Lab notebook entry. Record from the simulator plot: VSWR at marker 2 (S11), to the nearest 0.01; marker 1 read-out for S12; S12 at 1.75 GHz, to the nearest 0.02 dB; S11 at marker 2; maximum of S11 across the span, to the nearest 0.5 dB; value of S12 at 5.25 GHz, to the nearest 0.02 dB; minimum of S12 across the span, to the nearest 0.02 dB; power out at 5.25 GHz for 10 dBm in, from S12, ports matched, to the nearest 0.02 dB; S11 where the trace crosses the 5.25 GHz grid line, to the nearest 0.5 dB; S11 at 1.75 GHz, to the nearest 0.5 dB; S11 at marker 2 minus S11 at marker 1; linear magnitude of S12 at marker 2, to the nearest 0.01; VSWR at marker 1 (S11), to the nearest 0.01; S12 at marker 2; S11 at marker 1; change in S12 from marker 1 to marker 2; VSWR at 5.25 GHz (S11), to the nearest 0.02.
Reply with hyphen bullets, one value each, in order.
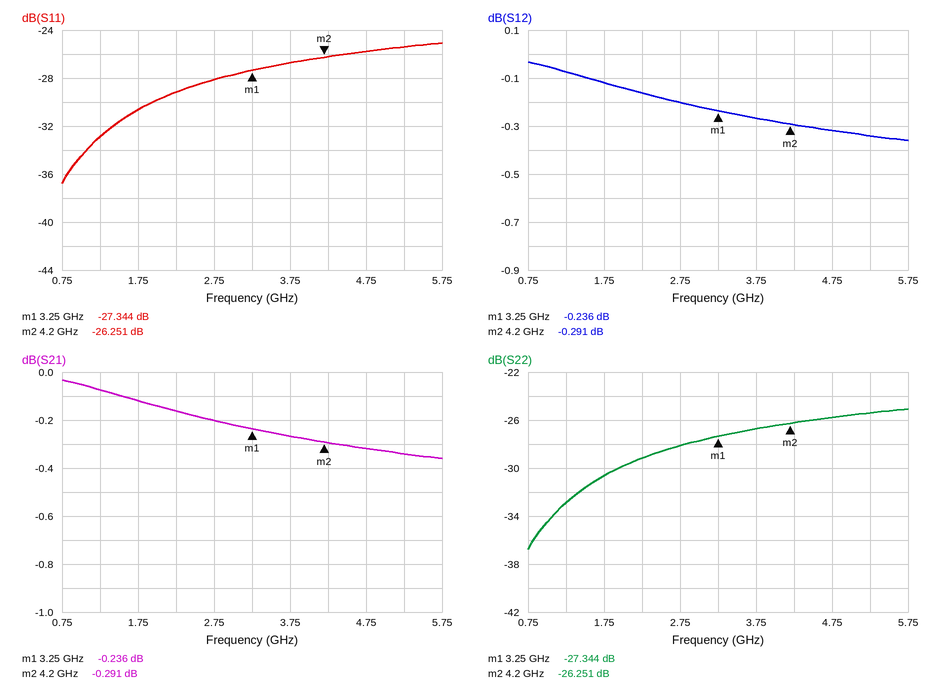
- 1.10
- -0.236 dB
- -0.12 dB
- -26.251 dB
- -25.0 dB
- -0.34 dB
- -0.36 dB
- 9.66 dBm
- -25.5 dB
- -30.5 dB
- 1.093 dB
- 0.97
- 1.09
- -0.291 dB
- -27.344 dB
- -0.055 dB
- 1.12
